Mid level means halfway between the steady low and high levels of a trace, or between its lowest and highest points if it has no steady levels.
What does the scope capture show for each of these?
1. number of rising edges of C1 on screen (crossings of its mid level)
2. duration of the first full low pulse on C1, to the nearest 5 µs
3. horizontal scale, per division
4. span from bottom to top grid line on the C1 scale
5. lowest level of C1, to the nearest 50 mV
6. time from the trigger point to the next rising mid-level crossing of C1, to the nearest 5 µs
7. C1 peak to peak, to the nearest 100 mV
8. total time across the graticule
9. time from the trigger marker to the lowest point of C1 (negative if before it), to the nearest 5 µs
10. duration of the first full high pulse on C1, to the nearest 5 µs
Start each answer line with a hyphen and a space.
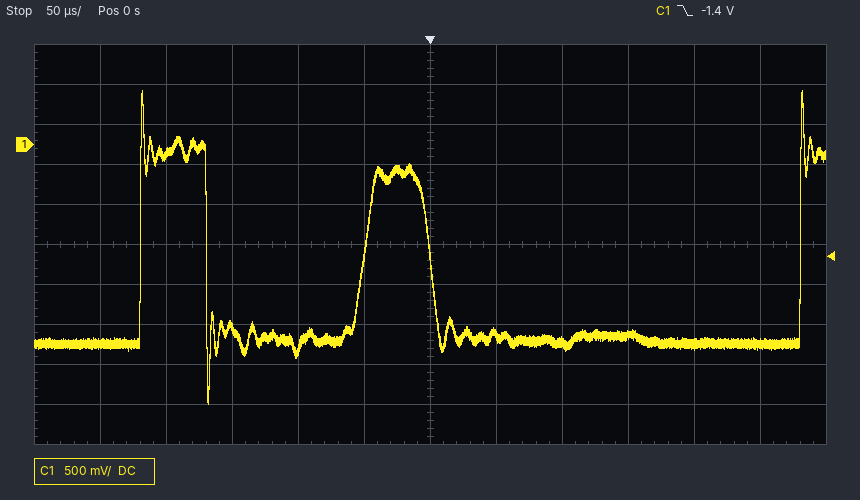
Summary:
- 3
- 120 µs
- 50 µs
- 5 V
- -3.25 V
- 280 µs
- 3.90 V
- 600 µs
- -170 µs
- 50 µs
